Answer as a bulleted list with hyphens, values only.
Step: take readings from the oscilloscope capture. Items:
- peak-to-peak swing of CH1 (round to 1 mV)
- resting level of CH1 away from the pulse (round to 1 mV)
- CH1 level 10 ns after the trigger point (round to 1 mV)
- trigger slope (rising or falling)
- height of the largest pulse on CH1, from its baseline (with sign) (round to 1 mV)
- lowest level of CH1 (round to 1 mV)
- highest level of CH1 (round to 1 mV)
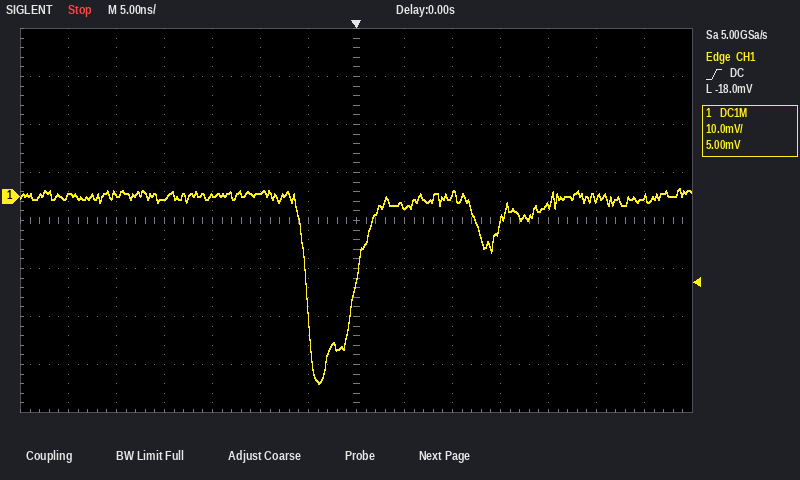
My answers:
- 41 mV
- 0 mV
- 0 mV
- rising
- -39 mV
- -39 mV
- 2 mV
